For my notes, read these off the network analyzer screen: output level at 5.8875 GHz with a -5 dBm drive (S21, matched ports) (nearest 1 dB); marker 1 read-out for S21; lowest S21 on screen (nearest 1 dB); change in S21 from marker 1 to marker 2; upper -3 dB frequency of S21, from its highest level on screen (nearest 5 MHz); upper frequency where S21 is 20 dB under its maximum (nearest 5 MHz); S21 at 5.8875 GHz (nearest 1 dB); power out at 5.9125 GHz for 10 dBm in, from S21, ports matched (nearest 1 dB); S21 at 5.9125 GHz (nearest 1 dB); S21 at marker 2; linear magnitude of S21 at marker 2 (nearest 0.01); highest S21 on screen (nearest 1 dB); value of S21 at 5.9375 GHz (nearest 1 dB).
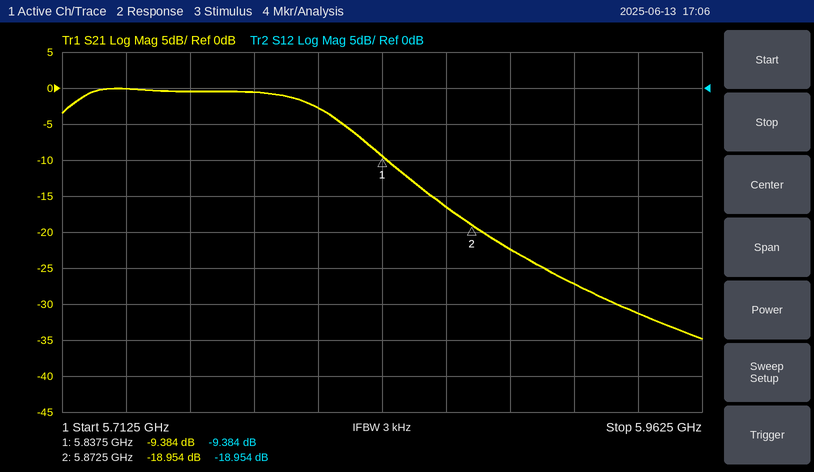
-27 dBm
-9.384 dB
-35 dB
-9.570 dB
5.815 GHz
5.875 GHz
-22 dB
-17 dBm
-27 dB
-18.954 dB
0.11
0 dB
-31 dB
